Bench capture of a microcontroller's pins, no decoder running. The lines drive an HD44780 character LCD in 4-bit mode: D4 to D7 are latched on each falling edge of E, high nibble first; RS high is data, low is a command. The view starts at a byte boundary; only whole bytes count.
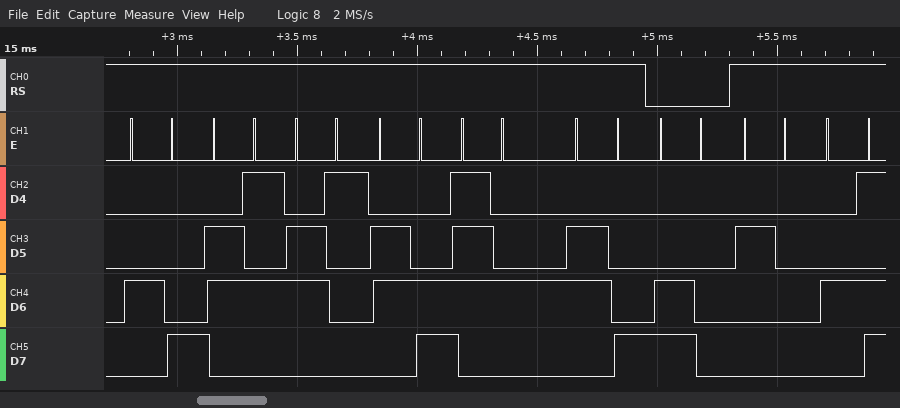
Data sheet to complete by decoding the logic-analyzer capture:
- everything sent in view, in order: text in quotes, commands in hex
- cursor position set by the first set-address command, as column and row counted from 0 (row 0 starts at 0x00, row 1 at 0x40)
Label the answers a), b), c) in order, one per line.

a) "Health" 0xC0 " M"
b) column 0, row 1
